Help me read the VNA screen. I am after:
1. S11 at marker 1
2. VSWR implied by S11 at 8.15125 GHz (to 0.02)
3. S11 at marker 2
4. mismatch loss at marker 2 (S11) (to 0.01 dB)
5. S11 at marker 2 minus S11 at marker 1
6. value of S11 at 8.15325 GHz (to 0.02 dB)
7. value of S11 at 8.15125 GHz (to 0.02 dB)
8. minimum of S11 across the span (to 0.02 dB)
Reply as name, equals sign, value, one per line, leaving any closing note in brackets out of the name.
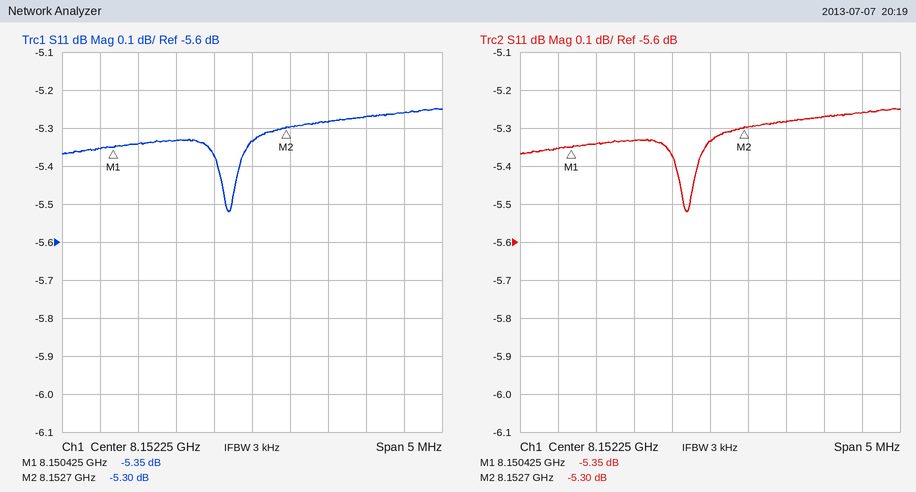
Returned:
S11 at marker 1 = -5.35 dB
VSWR implied by S11 at 8.15125 GHz = 3.36
S11 at marker 2 = -5.30 dB
mismatch loss at marker 2 (S11) = 1.52 dB
S11 at marker 2 minus S11 at marker 1 = 0.05 dB
value of S11 at 8.15325 GHz = -5.28 dB
value of S11 at 8.15125 GHz = -5.34 dB
minimum of S11 across the span = -5.52 dB
